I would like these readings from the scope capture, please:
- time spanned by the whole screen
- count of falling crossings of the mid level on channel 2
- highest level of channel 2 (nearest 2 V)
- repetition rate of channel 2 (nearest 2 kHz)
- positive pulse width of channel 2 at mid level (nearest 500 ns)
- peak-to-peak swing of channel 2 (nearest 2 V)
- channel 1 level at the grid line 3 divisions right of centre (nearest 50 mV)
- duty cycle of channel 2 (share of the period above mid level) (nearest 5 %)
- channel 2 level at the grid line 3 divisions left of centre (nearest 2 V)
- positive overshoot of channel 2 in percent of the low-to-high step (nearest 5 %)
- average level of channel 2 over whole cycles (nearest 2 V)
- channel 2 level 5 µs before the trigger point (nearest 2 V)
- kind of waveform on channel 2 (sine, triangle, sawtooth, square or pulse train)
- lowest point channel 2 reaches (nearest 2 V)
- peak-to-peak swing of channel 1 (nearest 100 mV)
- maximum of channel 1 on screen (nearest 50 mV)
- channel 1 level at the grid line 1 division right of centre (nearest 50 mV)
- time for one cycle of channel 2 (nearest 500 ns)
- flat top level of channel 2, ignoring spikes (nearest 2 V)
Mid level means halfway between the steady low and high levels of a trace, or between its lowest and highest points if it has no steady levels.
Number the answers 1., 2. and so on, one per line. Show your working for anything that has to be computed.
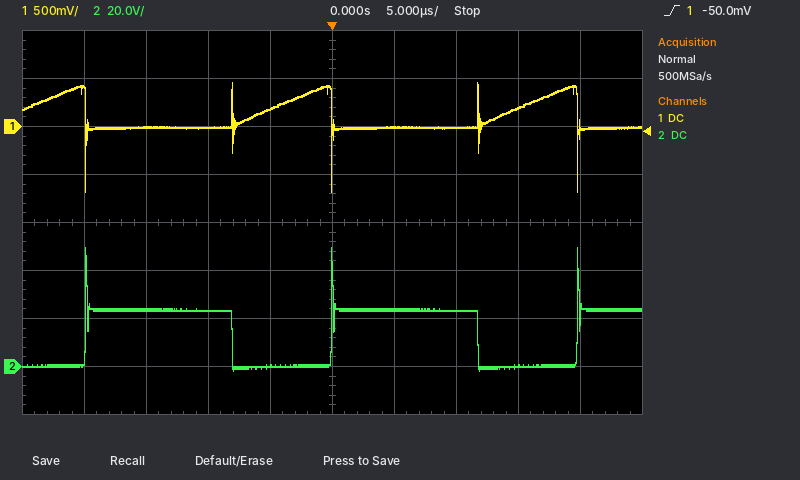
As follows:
1. 50 µs
2. 2
3. 50 V
4. 1 / 20.0 µs ≈ 50 kHz
5. 12.0 µs
6. 50 V − (-2 V) = 52 V
7. 200 mV
8. 12.0 µs / 20.0 µs ≈ 60 %
9. 24 V
10. 110 %
11. -2 V + 0.6 × (24 V − (-2 V)) ≈ 14 V
12. 0 V
13. pulse train
14. -2 V
15. 1.10 V
16. 450 mV
17. 0 mV
18. 20.0 µs
19. 24 V
